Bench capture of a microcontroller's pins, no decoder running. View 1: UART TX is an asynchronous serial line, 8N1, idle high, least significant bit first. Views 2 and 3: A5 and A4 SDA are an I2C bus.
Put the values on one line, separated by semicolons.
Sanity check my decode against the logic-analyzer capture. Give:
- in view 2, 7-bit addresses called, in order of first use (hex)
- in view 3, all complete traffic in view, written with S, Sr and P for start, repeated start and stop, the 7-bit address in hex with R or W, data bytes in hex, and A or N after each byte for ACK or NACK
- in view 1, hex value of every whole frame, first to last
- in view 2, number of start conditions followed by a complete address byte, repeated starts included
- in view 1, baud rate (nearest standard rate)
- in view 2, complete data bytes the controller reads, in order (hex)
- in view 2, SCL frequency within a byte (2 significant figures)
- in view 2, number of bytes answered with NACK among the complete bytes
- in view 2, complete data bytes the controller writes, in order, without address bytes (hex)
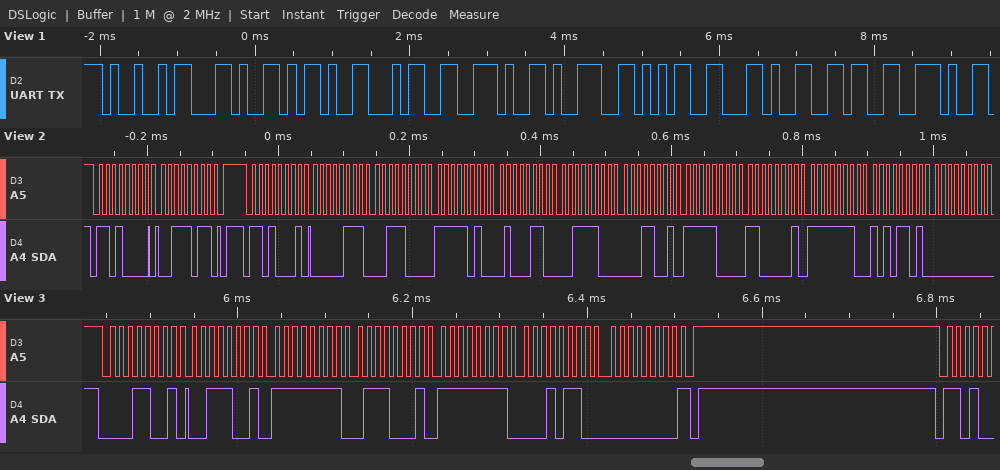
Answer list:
0x68; S 0CR A 39 A FF A 71 A FF A 16 A 00 N P; 49 2C 2D 34 2E 39 35 2C 36 2E; 2; 9600 baud; 07 38 FA 46 3C 19 F8 C1 FE AD 00; 100 kHz; 0; 3B
